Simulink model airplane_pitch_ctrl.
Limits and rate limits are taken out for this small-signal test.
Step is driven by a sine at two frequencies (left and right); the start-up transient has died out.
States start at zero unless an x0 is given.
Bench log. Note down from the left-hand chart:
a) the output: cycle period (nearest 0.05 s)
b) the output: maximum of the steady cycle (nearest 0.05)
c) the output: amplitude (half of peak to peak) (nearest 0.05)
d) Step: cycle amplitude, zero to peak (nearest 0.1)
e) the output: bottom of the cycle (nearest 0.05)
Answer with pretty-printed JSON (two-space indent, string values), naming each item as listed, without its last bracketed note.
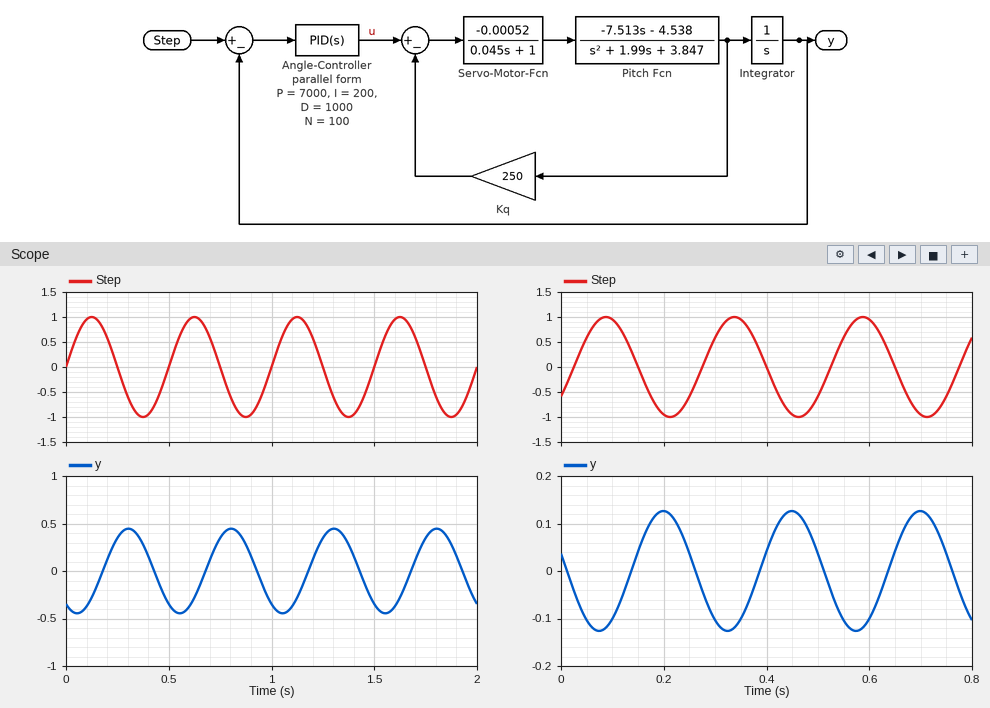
{
  "the output: cycle period": "0.50 s",
  "the output: maximum of the steady cycle": "0.45",
  "the output: amplitude (half of peak to peak)": "0.45",
  "Step: cycle amplitude, zero to peak": "1.0",
  "the output: bottom of the cycle": "-0.45"
}
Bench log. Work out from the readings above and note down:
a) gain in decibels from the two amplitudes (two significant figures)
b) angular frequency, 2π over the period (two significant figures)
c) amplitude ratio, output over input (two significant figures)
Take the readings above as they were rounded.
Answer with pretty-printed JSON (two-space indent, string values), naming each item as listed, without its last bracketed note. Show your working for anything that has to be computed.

{
  "gain in decibels from the two amplitudes": "20 log10(0.45 / 1) = -6.9 dB",
  "angular frequency, 2π over the period": "2π / 0.5 = 13 rad/s",
  "amplitude ratio, output over input": "0.45 / 1 = 0.45"
}
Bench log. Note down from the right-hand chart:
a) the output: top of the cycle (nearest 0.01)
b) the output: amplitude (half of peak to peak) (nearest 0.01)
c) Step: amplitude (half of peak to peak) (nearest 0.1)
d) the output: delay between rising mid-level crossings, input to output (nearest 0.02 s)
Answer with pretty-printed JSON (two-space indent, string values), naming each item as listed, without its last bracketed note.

{
  "the output: top of the cycle": "0.13",
  "the output: amplitude (half of peak to peak)": "0.13",
  "Step: amplitude (half of peak to peak)": "1.0",
  "the output: delay between rising mid-level crossings, input to output": "0.12 s"
}
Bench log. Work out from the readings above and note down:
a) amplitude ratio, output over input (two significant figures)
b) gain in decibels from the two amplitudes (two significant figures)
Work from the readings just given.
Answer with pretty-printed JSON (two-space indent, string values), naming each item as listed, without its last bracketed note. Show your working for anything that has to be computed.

{
  "amplitude ratio, output over input": "0.13 / 1 = 0.13",
  "gain in decibels from the two amplitudes": "20 log10(0.13 / 1) = -18 dB"
}
